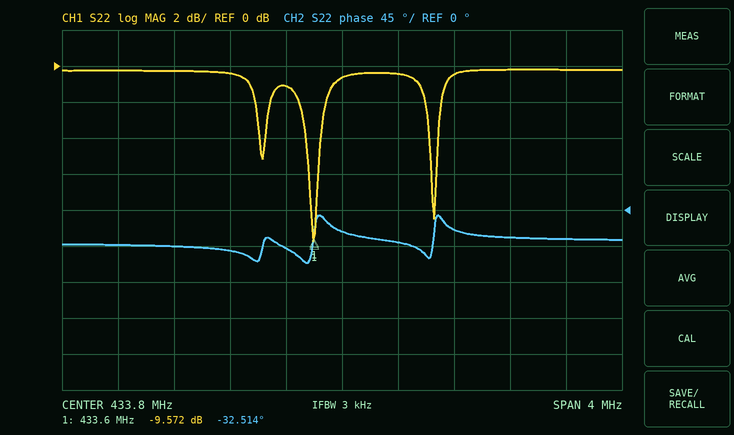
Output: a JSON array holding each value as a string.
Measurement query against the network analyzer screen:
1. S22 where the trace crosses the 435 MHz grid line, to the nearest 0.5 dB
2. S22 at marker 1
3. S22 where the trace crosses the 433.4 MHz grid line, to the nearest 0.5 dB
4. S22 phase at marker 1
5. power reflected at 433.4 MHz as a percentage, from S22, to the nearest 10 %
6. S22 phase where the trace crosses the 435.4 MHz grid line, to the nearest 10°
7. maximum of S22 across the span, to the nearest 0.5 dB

["0.0 dB", "-9.572 dB", "-1.0 dB", "-32.514°", "80 %", "-40°", "0.0 dB"]
